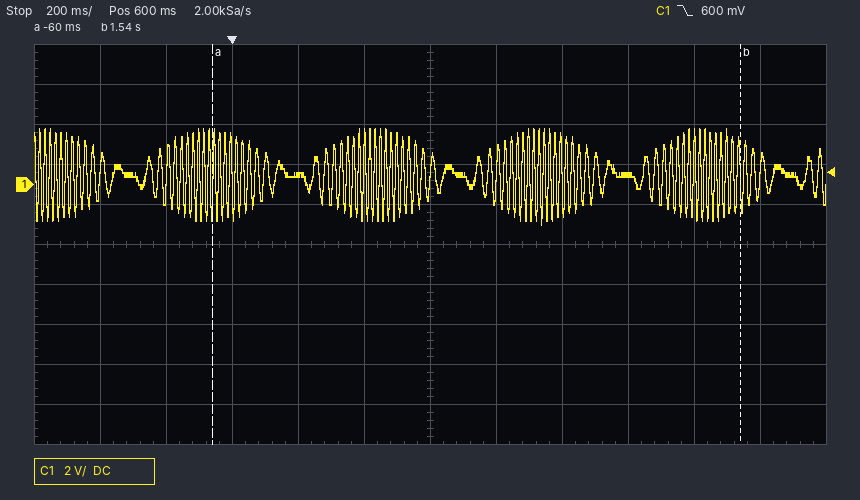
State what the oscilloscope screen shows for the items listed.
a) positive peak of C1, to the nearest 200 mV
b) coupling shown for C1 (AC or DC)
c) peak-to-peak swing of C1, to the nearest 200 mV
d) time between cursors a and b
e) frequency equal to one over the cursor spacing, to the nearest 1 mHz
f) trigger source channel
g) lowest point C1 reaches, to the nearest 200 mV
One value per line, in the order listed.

2.8 V
DC
4.8 V
1.60 s
625 mHz
C1
-2.0 V
